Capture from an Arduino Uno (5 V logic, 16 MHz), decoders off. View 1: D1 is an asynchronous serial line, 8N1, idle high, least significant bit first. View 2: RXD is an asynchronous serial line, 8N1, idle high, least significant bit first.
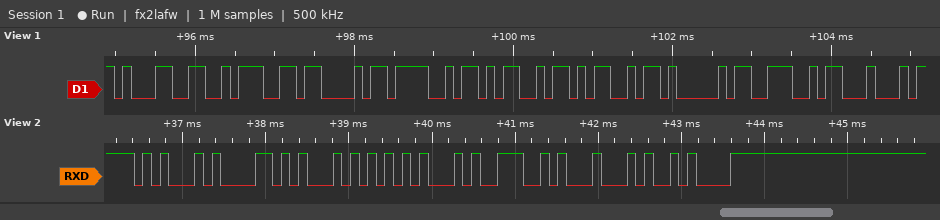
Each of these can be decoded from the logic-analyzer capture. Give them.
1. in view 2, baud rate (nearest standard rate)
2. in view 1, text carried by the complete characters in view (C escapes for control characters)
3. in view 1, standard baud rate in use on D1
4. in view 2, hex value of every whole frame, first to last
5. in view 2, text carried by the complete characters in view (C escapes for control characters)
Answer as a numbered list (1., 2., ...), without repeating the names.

1. 9600 baud
2. "1:COMMAND"
3. 9600 baud
4. 0x45 0x58 0x54 0x45 0x4E 0x44 0x0A
5. "EXTEND\n"
